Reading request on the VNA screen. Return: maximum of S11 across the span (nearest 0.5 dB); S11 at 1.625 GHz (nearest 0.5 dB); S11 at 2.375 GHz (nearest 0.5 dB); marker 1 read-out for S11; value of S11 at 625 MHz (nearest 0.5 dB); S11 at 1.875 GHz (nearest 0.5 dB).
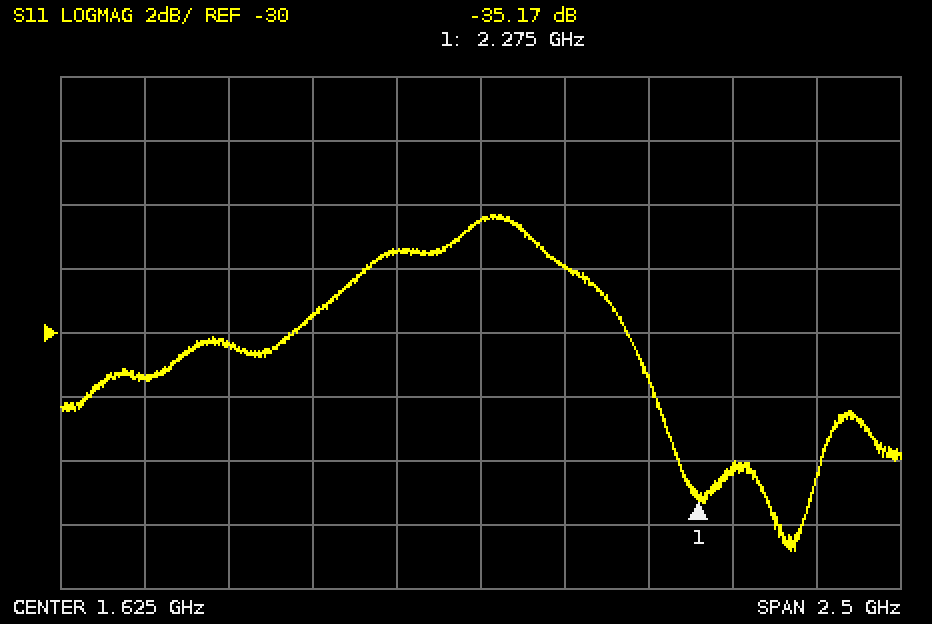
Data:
-26.5 dB
-26.5 dB
-34.5 dB
-35.17 dB
-31.5 dB
-28.0 dB
